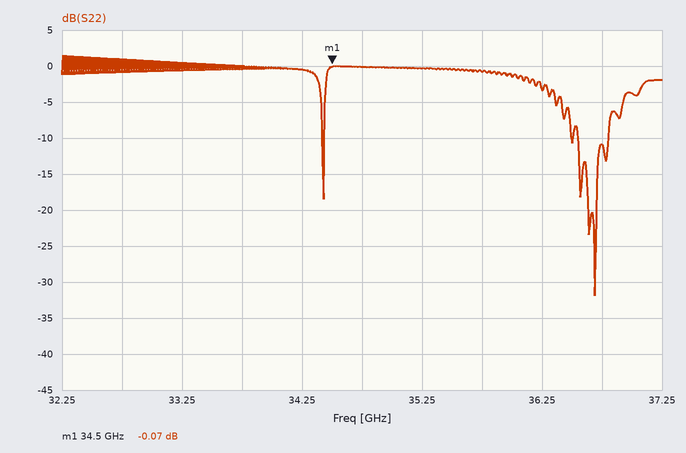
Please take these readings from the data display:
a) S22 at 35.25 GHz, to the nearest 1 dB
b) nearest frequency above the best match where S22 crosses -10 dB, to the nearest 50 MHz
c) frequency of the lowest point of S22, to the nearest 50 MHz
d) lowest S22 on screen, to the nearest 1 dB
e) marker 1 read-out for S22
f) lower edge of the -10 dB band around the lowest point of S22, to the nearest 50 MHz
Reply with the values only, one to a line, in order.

0 dB
36.80 GHz
36.70 GHz
-32 dB
-0.07 dB
36.55 GHz
